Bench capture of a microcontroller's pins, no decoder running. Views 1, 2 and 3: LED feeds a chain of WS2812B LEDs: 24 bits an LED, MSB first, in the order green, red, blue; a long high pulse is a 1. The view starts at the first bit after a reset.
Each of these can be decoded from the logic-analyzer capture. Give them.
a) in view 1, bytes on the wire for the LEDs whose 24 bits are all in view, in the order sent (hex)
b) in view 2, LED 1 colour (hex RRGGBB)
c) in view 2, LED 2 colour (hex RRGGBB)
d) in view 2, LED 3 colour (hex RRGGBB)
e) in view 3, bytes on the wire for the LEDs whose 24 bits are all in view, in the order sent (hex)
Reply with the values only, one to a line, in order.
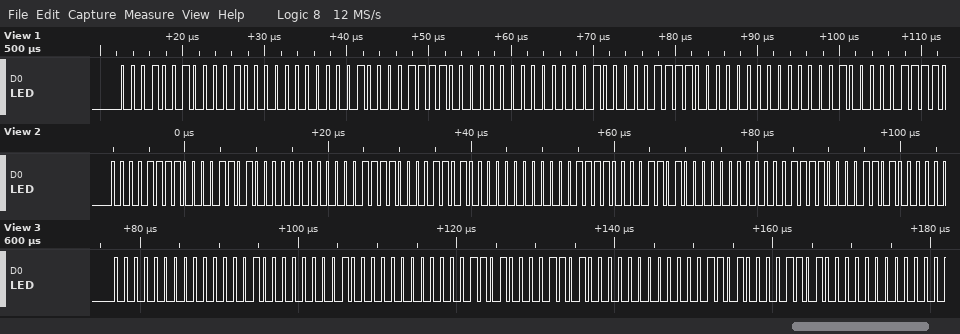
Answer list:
12 10 01 0F 00 02 0F 00 02
#0D0F00
#0D0F00
#0D0F00
00 02 01 00 0D 0D 00 0D 0D
